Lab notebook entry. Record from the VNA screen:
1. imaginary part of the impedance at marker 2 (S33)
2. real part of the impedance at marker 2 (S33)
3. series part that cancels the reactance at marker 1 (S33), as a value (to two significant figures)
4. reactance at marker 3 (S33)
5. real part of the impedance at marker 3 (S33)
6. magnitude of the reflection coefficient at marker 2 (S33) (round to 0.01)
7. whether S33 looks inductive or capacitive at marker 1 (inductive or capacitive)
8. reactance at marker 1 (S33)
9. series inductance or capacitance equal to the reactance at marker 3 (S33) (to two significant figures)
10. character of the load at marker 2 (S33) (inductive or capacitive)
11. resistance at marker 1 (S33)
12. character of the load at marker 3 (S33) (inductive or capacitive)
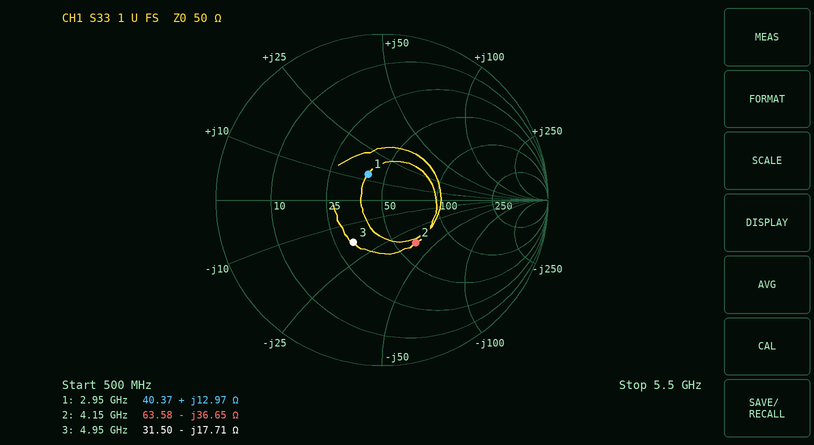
-36.65 Ω
63.58 Ω
4.2 pF
-17.71 Ω
31.50 Ω
0.33
inductive
+12.97 Ω
1.8 pF
capacitive
40.37 Ω
capacitive
